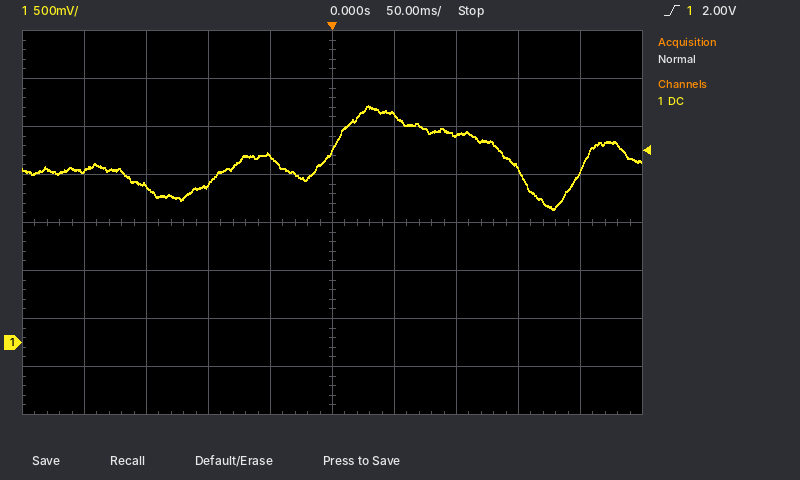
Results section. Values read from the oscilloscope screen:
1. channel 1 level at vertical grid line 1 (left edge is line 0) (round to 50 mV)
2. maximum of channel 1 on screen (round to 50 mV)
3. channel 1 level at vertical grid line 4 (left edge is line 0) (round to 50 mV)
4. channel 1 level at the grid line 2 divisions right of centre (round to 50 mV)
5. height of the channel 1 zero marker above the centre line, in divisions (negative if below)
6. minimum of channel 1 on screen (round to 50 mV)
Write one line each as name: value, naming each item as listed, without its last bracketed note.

channel 1 level at vertical grid line 1 (left edge is line 0): 1.80 V
maximum of channel 1 on screen: 2.45 V
channel 1 level at vertical grid line 4 (left edge is line 0): 1.95 V
channel 1 level at the grid line 2 divisions right of centre: 2.15 V
height of the channel 1 zero marker above the centre line, in divisions: -2.5 div
minimum of channel 1 on screen: 1.40 V
